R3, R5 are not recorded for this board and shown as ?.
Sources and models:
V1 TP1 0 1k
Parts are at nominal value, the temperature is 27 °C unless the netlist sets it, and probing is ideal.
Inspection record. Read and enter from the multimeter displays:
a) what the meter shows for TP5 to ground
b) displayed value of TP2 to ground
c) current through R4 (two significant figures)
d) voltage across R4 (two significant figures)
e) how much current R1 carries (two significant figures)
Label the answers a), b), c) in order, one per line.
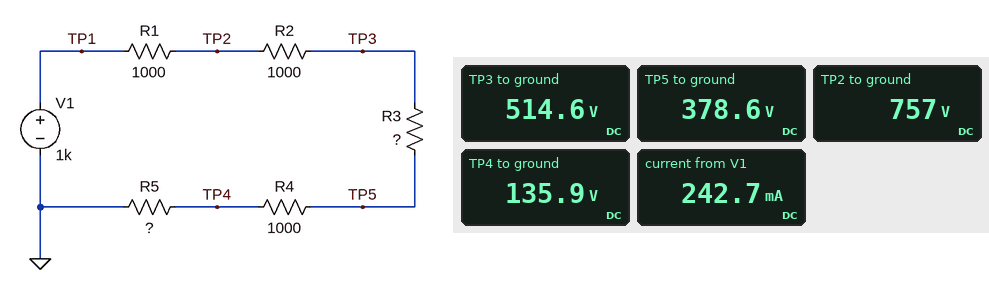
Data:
a) 378.6 V
b) 757 V
c) 240 mA
d) 240 V
e) 240 mA
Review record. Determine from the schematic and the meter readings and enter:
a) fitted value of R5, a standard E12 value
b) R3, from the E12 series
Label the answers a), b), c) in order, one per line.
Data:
a) 560 Ω
b) 560 Ω
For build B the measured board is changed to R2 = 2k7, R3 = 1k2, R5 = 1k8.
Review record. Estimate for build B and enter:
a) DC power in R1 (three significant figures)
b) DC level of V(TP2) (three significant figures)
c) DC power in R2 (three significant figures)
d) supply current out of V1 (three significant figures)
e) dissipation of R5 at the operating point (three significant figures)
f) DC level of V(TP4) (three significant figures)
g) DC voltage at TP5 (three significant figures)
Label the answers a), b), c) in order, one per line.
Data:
a) 16.9 W
b) 870 V
c) 45.5 W
d) 130 mA
e) 30.4 W
f) 234 V
g) 364 V
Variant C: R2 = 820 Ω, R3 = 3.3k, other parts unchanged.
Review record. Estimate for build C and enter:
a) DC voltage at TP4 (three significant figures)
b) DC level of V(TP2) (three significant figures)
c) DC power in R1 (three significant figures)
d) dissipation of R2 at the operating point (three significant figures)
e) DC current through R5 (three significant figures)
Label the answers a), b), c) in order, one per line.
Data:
a) 83.8 V
b) 850 V
c) 22.4 W
d) 18.4 W
e) 150 mA
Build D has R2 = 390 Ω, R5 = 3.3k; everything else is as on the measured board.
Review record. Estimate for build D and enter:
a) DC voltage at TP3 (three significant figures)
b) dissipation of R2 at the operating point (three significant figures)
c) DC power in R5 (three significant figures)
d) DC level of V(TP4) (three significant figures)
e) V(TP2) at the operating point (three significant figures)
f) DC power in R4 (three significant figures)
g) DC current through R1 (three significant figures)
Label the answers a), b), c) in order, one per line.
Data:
a) 778 V
b) 9.98 W
c) 84.5 W
d) 528 V
e) 840 V
f) 25.6 W
g) 160 mA
